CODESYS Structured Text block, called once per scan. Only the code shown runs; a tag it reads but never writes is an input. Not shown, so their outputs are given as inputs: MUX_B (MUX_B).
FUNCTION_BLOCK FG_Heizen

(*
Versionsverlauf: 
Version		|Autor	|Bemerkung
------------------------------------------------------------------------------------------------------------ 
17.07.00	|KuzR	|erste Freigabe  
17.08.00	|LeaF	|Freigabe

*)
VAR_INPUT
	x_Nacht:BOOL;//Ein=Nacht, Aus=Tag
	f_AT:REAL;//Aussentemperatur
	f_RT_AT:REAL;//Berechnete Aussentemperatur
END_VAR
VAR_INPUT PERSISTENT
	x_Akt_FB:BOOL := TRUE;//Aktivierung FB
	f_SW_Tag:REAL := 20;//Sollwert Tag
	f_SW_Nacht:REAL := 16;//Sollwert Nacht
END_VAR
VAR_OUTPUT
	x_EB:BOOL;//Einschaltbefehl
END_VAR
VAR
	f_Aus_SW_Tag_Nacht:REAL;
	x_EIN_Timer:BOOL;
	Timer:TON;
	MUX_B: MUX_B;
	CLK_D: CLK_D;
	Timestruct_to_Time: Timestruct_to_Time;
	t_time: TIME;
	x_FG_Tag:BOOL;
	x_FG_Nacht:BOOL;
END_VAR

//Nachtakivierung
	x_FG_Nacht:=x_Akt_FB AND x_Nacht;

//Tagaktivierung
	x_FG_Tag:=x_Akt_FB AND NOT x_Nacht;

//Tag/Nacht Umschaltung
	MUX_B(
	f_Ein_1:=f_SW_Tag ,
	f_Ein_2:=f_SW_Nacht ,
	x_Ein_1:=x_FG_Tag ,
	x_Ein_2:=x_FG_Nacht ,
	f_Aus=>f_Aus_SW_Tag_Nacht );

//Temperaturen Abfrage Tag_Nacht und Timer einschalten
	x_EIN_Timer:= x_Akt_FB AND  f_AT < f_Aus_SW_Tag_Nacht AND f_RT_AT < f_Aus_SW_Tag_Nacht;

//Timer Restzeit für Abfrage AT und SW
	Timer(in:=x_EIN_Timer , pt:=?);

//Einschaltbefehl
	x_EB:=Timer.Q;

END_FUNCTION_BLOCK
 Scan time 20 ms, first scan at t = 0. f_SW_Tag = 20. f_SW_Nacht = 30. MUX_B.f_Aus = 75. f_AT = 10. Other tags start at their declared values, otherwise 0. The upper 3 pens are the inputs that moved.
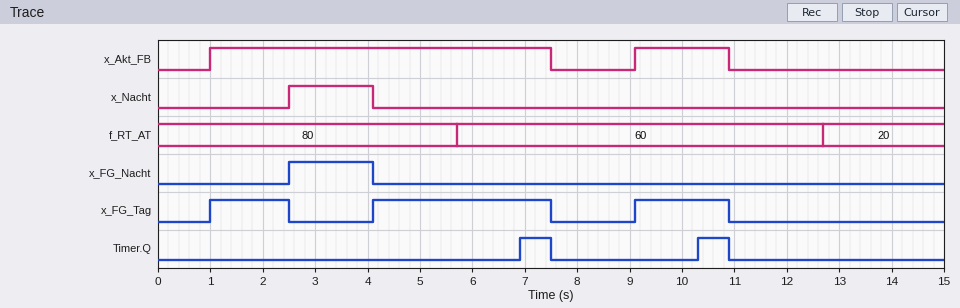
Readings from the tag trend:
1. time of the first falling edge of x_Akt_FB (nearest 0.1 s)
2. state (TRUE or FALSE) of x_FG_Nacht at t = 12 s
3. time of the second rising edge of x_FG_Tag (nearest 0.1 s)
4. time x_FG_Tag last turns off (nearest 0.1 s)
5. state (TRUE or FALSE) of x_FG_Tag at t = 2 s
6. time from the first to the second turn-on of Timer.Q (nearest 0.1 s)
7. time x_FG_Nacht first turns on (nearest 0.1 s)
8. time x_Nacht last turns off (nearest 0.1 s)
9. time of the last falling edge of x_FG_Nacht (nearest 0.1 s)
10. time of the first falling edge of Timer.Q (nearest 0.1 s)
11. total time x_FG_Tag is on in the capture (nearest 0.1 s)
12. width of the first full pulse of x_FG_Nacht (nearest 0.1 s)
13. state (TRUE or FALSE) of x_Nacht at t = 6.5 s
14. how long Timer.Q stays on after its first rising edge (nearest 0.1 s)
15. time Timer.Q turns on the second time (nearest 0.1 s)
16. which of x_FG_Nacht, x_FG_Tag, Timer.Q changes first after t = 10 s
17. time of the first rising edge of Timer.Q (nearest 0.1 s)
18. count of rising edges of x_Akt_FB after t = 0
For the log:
7.5 s
FALSE
4.1 s
10.9 s
TRUE
3.4 s
2.5 s
4.1 s
4.1 s
7.5 s
6.7 s
1.6 s
FALSE
0.6 s
10.3 s
Timer.Q
6.9 s
2
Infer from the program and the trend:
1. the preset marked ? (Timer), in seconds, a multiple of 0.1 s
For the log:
1.2 s
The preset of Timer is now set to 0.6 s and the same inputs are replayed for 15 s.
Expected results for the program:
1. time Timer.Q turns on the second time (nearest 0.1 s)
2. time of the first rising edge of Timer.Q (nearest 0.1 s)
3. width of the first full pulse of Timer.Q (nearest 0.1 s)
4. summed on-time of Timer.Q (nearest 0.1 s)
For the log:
9.7 s
6.3 s
1.2 s
2.4 s
